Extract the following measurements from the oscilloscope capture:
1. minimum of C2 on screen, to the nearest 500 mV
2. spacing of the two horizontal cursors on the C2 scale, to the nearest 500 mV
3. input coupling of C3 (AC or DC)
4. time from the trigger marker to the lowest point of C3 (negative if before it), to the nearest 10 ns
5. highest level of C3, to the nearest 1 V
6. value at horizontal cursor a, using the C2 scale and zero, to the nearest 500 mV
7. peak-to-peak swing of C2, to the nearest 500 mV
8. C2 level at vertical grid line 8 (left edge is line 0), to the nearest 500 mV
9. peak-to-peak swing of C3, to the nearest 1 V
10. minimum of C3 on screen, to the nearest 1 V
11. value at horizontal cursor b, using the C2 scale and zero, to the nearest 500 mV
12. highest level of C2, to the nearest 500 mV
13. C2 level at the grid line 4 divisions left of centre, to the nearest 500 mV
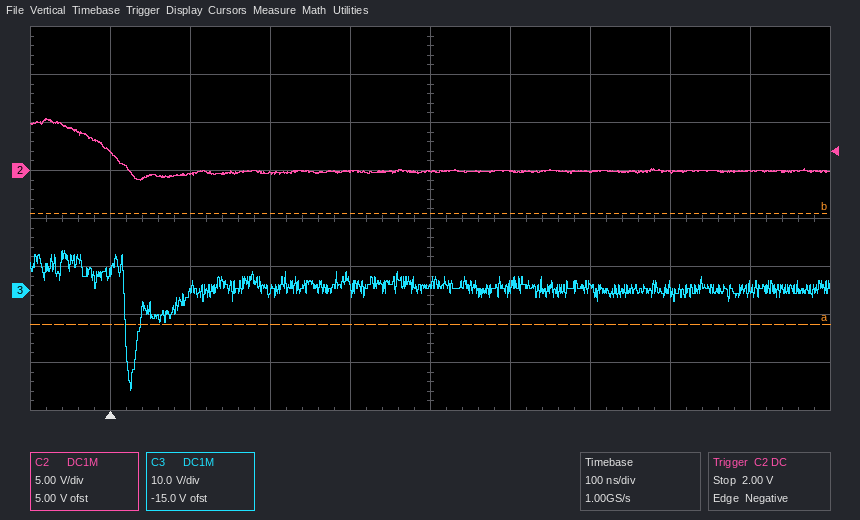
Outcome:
-1.0 V
11.5 V
DC
+30 ns
8 V
-16.0 V
6.5 V
0.0 V
29 V
-21 V
-4.5 V
5.5 V
2.0 V
